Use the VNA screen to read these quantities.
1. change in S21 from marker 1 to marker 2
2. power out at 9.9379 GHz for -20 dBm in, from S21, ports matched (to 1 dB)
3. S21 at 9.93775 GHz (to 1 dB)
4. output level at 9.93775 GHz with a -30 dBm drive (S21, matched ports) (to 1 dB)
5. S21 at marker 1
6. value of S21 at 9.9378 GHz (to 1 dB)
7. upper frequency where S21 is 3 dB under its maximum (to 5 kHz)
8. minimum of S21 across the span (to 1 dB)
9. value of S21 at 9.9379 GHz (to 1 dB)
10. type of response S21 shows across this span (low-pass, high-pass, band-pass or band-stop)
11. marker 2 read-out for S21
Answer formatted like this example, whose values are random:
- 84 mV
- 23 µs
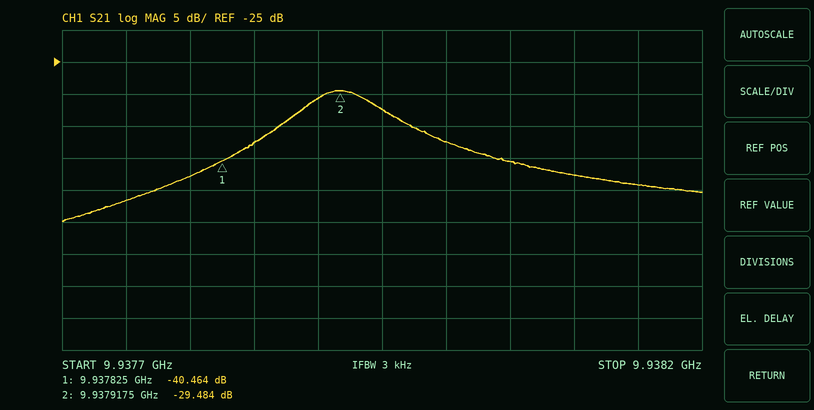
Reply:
- 10.980 dB
- -51 dBm
- -47 dB
- -77 dBm
- -40.464 dB
- -43 dB
- 9.937950 GHz
- -50 dB
- -31 dB
- band-pass
- -29.484 dB
